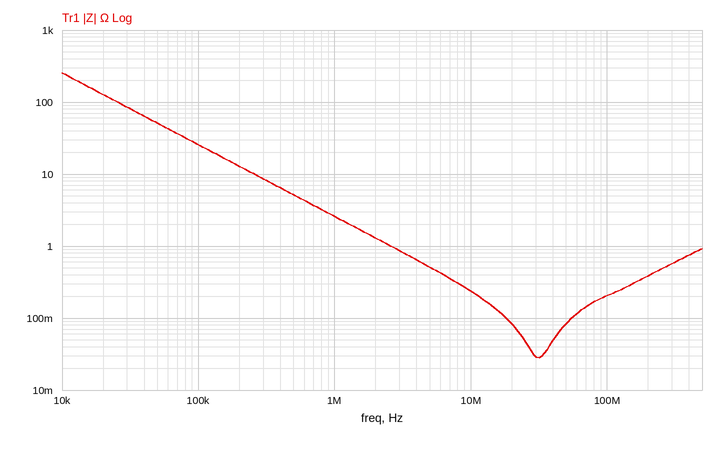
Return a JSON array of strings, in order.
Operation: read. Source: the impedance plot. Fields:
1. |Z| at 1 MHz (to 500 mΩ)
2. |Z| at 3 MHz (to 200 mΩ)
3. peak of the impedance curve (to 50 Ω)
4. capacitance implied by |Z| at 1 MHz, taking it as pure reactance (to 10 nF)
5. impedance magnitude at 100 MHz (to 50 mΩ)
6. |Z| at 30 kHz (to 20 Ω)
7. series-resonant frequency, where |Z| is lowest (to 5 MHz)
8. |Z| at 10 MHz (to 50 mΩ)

["2.5 Ω", "800 mΩ", "250 Ω", "60 nF", "200 mΩ", "80 Ω", "30 MHz", "250 mΩ"]
